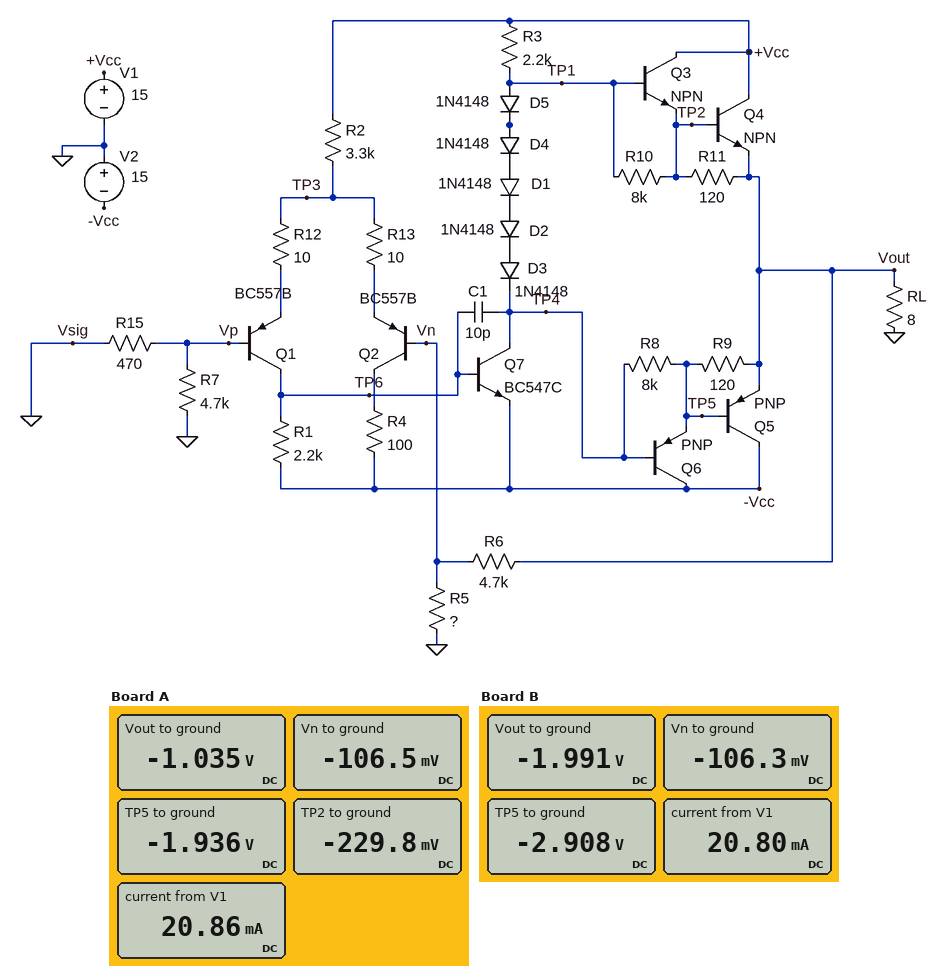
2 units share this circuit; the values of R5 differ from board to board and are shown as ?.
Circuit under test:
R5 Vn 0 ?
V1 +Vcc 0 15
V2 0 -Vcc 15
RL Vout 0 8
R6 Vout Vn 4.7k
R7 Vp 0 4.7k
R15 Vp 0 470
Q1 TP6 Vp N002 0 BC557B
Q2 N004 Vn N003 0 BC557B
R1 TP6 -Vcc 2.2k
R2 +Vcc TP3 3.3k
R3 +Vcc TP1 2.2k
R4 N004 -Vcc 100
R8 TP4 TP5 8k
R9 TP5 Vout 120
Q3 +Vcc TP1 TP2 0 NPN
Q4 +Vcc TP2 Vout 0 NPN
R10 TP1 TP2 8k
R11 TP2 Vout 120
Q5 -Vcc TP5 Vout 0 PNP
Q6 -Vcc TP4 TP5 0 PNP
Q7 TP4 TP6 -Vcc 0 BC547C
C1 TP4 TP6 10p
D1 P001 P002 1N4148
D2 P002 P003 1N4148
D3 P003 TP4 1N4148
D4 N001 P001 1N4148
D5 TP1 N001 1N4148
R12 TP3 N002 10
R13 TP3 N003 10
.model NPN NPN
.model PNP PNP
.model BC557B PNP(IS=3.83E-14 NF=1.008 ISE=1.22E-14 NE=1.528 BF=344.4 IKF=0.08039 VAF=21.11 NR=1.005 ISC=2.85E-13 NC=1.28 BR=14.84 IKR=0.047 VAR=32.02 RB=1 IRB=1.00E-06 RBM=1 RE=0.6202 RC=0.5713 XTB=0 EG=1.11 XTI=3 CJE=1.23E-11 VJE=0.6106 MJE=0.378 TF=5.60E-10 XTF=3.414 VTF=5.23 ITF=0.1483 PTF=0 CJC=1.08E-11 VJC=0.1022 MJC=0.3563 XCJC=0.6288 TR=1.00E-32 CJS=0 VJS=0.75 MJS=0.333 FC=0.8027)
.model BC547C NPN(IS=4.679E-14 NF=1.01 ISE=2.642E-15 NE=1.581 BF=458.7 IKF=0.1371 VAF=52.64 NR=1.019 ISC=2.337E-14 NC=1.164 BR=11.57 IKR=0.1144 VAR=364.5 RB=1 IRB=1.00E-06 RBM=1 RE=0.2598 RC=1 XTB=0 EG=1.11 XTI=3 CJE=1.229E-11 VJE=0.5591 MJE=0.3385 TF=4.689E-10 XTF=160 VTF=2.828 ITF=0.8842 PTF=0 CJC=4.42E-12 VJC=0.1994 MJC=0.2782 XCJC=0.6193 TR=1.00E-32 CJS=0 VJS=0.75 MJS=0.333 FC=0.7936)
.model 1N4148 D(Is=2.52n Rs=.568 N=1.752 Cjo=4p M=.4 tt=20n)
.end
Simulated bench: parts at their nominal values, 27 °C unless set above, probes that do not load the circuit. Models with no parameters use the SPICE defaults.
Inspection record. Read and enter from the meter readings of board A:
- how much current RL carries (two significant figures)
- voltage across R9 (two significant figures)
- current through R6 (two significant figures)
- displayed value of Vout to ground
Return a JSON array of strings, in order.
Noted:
["130 mA", "900 mV", "200 µA", "-1.035 V"]
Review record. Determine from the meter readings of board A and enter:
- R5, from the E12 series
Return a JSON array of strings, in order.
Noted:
["560 Ω"]
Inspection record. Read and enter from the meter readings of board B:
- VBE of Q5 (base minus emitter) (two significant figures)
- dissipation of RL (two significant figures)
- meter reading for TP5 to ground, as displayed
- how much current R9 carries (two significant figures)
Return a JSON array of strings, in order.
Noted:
["-920 mV", "500 mW", "-2.908 V", "7.6 mA"]
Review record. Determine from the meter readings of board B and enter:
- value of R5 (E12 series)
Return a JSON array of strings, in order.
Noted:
["270 Ω"]
